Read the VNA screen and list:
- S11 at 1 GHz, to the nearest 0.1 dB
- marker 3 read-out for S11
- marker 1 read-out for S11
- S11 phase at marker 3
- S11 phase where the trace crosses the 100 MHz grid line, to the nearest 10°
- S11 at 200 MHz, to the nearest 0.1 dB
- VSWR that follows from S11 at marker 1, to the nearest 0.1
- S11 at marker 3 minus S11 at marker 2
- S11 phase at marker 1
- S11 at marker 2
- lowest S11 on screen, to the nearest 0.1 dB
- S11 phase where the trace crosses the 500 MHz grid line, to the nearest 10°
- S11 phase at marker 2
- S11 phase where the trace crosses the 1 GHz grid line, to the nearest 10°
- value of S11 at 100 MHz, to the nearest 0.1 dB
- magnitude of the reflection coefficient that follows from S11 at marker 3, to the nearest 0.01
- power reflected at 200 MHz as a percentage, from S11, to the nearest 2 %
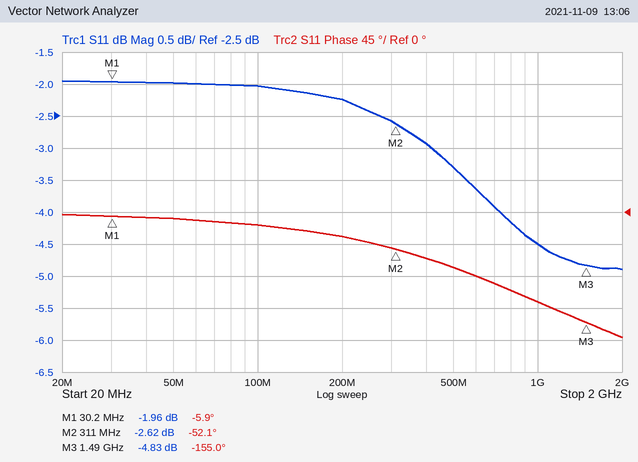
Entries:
-4.5 dB
-4.83 dB
-1.96 dB
-155.0°
-20°
-2.2 dB
8.9
-2.21 dB
-5.9°
-2.62 dB
-4.9 dB
-80°
-52.1°
-130°
-2.0 dB
0.57
60 %
